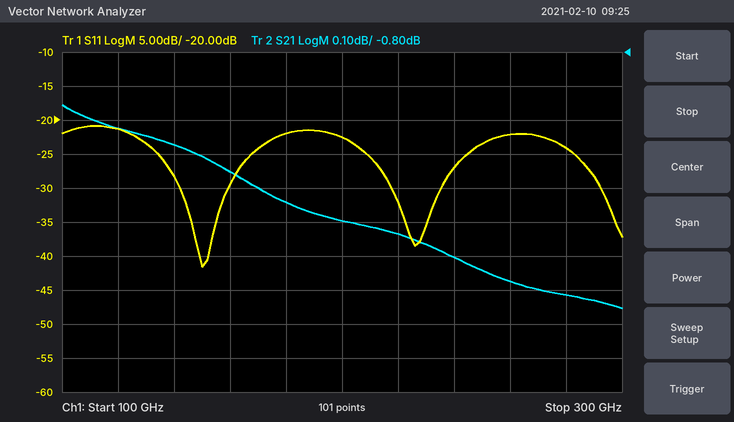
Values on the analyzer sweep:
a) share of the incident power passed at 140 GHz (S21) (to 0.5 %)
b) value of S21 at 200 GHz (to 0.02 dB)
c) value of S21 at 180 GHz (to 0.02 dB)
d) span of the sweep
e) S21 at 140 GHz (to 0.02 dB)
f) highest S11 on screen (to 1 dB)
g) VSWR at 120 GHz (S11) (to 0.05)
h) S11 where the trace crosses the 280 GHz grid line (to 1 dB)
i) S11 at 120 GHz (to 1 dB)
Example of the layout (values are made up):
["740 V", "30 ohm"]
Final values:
["78.0 %", "-1.30 dB", "-1.24 dB", "200 GHz", "-1.08 dB", "-21 dB", "1.20", "-24 dB", "-21 dB"]
